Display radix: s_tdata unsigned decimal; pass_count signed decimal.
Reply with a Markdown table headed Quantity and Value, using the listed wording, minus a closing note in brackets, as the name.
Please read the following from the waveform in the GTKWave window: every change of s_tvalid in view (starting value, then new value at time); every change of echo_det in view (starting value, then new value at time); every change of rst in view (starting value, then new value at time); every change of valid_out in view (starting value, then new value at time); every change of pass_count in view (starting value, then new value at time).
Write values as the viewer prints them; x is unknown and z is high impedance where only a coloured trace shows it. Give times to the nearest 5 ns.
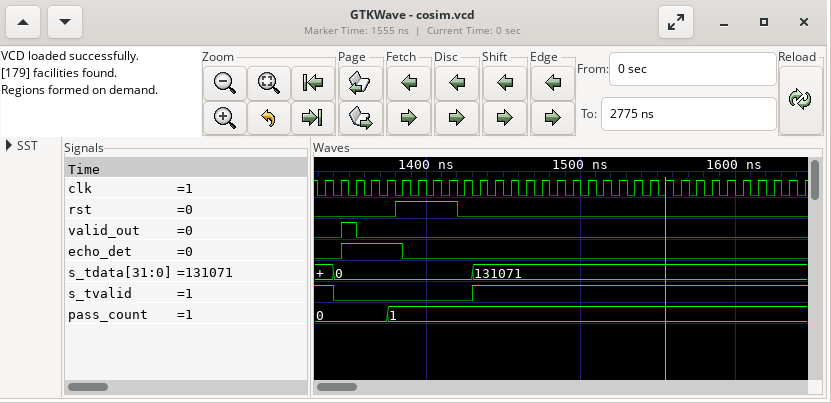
| Quantity | Value |
|---|---|
| every change of s_tvalid in view | 1, 0 at 1340 ns, 1 at 1430 ns |
| every change of echo_det in view | 0, 1 at 1345 ns, 0 at 1385 ns |
| every change of rst in view | 0, 1 at 1380 ns, 0 at 1420 ns |
| every change of valid_out in view | 0, 1 at 1345 ns, 0 at 1355 ns |
| every change of pass_count in view | 0, 1 at 1375 ns |
